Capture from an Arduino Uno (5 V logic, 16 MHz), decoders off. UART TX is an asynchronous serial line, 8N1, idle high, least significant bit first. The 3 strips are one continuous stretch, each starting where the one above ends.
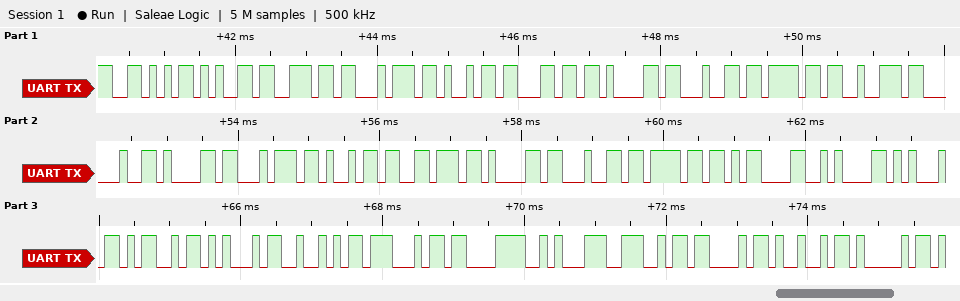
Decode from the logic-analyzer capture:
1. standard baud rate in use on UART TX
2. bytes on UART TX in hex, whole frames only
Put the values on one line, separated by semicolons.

9600 baud; 56 65 6E 74 69 6C 61 64 6F 72 20 61 74 69 76 61 64 6F 0D 0A 45 4D 45 52 47 C3 8A 4E 43 49 41
